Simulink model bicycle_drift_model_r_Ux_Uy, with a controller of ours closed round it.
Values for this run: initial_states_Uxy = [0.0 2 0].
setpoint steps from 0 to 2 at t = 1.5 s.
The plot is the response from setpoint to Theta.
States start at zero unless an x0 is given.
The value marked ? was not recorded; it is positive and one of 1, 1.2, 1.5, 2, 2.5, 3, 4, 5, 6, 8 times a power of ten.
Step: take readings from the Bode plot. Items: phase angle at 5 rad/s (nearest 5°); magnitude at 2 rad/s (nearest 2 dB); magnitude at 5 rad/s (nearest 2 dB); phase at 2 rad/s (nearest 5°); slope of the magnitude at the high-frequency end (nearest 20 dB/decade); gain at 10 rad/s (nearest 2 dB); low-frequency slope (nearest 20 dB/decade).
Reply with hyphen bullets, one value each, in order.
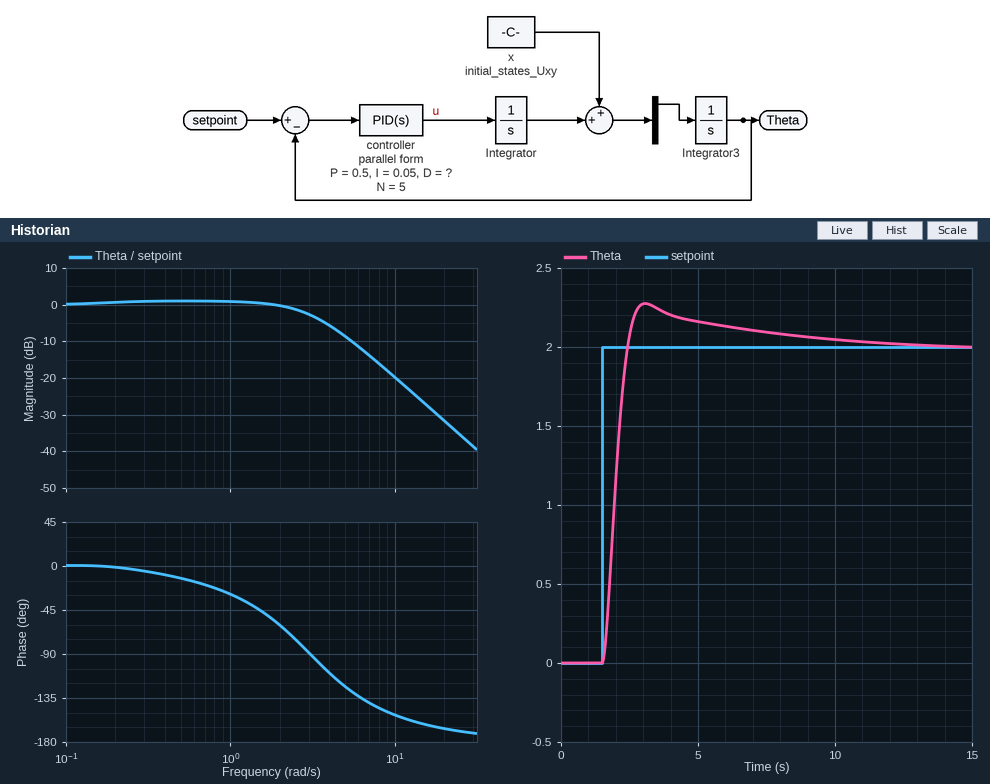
- -125°
- 0 dB
- -8 dB
- -60°
- -40 dB/decade
- -20 dB
- 0 dB/decade
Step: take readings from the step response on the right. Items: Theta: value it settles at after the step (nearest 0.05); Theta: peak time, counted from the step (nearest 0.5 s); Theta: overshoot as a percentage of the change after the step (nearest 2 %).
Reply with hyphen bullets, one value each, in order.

- 2.00
- 1.5 s
- 14 %
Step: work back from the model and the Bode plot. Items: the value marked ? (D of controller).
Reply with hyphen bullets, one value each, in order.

- 2
